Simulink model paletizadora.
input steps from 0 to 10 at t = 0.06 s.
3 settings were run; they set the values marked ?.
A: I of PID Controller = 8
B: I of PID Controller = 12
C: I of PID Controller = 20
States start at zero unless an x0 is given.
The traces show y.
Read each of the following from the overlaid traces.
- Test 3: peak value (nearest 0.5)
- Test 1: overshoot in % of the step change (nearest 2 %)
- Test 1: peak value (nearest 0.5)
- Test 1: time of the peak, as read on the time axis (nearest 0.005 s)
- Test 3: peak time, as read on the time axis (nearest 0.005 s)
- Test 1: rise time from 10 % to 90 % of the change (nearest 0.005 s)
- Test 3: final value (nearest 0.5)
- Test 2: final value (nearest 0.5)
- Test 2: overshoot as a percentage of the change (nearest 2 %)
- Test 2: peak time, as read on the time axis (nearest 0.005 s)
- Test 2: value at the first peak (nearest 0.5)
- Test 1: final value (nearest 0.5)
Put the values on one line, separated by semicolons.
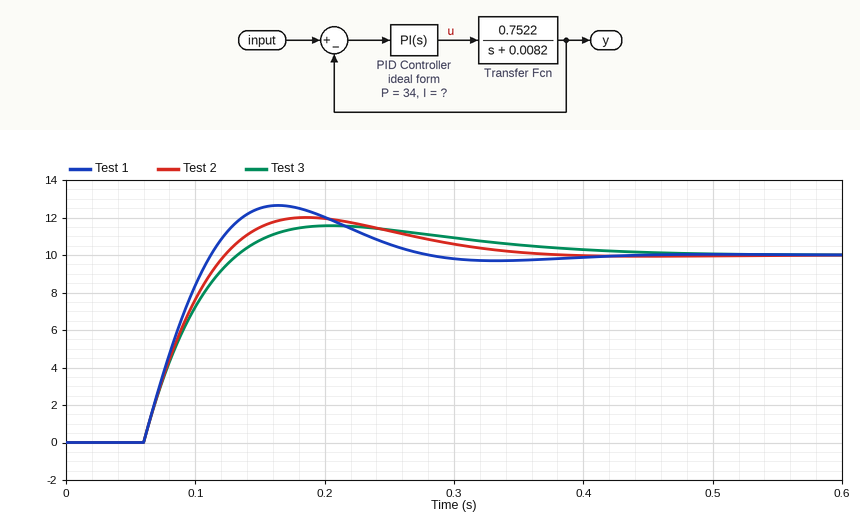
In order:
11.5; 26 %; 12.5; 0.165 s; 0.205 s; 0.040 s; 10.0; 10.0; 20 %; 0.185 s; 12.0; 10.0
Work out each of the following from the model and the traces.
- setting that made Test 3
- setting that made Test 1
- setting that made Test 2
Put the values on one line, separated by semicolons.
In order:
A; C; B
